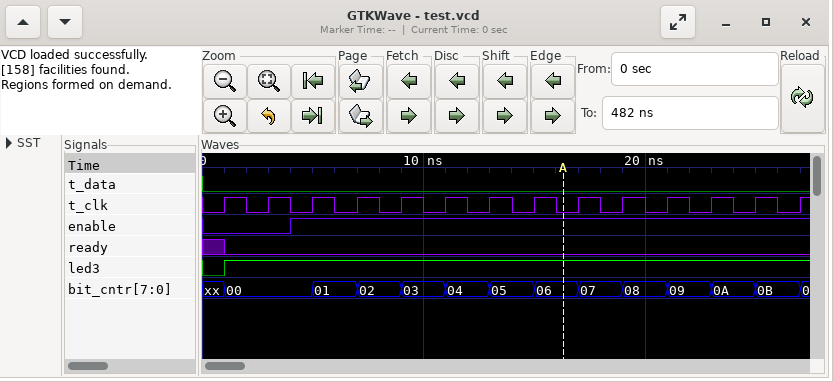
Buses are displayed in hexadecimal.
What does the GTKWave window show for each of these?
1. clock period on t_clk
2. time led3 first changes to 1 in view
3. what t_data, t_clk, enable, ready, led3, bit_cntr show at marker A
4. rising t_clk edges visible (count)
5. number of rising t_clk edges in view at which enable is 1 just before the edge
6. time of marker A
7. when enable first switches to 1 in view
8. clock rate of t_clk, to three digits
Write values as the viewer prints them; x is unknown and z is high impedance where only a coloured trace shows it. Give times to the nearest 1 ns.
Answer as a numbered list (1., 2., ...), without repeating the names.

1. 2 ns
2. 1 ns
3. t_data=0, t_clk=0, enable=1, ready=0, led3=1, bit_cntr=06
4. 14
5. 12
6. 16 ns
7. 4 ns
8. 500 MHz
